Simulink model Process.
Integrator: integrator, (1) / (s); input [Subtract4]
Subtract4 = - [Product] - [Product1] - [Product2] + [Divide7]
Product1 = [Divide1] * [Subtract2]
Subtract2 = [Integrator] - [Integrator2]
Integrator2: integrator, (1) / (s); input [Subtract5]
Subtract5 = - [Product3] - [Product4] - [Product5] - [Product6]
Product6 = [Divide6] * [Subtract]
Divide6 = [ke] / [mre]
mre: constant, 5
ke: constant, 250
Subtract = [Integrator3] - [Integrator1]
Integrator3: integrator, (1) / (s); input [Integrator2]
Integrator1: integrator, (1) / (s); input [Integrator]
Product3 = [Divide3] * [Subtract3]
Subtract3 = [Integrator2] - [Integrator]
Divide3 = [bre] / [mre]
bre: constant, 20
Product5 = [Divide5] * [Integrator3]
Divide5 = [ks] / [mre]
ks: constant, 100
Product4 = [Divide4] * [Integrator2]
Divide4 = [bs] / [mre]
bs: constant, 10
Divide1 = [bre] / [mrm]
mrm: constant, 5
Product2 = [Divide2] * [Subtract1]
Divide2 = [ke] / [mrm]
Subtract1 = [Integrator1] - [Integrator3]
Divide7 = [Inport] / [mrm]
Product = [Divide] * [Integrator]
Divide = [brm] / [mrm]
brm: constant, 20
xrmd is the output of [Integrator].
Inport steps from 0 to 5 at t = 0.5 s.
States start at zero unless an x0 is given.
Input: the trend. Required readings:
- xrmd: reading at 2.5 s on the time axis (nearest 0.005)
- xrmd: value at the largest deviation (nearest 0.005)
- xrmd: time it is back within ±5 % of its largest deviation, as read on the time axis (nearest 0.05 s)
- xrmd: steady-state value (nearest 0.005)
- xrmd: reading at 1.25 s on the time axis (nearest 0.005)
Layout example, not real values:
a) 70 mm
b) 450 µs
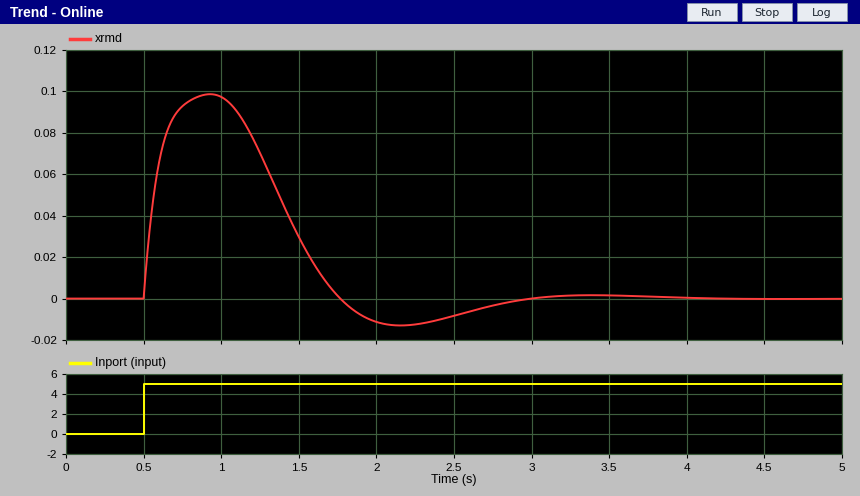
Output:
a) -0.010
b) 0.100
c) 2.65 s
d) 0.000
e) 0.070
